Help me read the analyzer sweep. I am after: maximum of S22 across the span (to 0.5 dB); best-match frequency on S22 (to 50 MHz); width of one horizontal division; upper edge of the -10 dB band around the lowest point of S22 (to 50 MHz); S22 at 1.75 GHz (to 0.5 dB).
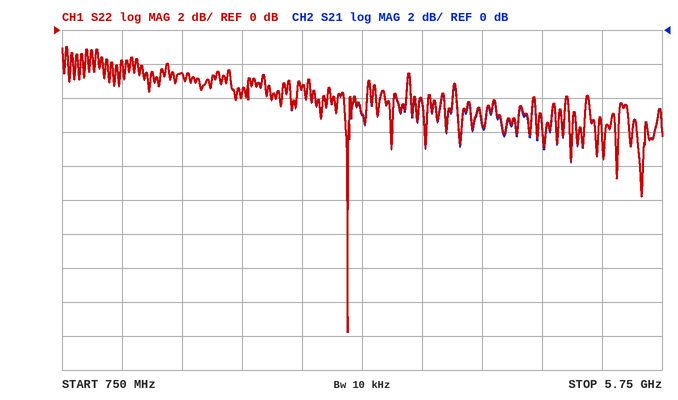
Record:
-1.0 dB
3.15 GHz
500 MHz
3.15 GHz
-2.5 dB
